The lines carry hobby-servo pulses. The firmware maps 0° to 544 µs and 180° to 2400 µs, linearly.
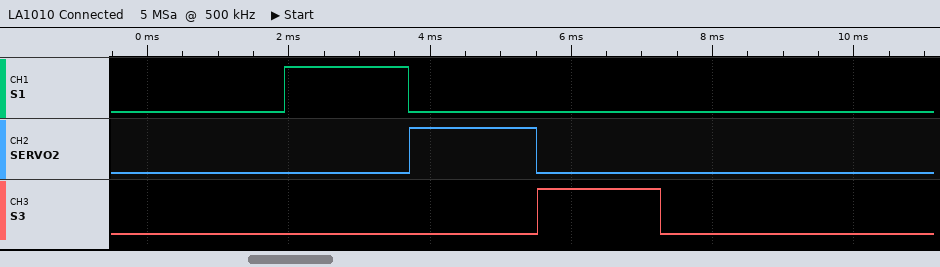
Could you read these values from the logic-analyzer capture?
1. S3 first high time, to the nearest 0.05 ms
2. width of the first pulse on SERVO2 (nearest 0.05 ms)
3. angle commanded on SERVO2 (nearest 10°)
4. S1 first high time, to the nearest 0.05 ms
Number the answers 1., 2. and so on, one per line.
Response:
1. 1.75 ms
2. 1.80 ms
3. 120°
4. 1.75 ms
